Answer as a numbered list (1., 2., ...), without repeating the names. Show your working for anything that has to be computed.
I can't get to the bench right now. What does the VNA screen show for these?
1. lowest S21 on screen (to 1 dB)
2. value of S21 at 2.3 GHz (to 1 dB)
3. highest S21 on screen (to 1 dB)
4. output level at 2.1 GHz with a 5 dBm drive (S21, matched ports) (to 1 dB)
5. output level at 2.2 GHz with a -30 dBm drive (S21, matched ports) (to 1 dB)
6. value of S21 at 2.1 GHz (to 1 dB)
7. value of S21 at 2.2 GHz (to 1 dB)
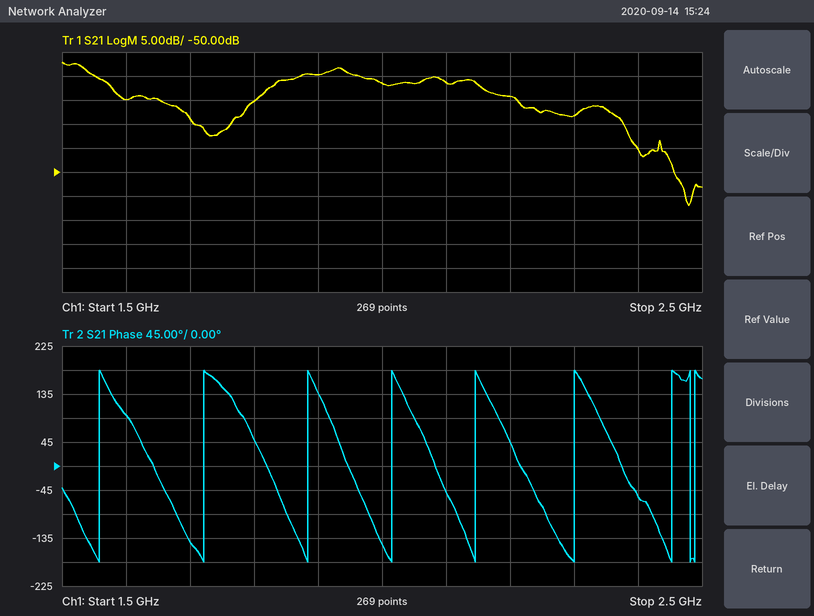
1. -57 dB
2. -38 dB
3. -27 dB
4. 5 dBm + (-31 dB) = -26 dBm
5. -30 dBm + (-34 dB) = -64 dBm
6. -31 dB
7. -34 dB
